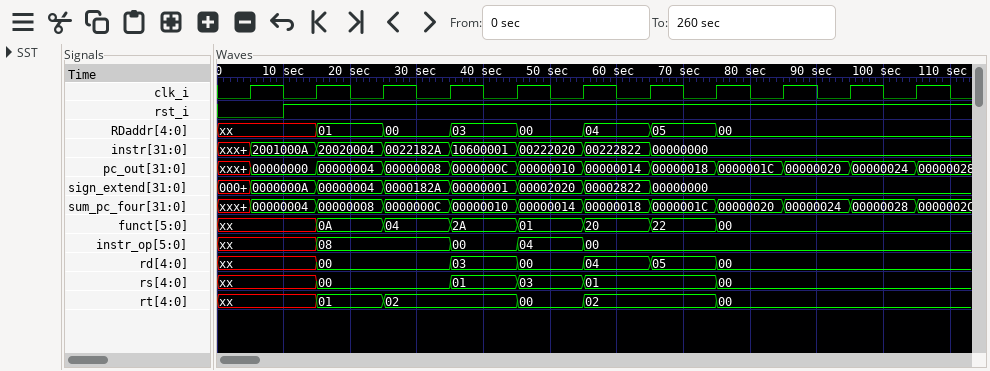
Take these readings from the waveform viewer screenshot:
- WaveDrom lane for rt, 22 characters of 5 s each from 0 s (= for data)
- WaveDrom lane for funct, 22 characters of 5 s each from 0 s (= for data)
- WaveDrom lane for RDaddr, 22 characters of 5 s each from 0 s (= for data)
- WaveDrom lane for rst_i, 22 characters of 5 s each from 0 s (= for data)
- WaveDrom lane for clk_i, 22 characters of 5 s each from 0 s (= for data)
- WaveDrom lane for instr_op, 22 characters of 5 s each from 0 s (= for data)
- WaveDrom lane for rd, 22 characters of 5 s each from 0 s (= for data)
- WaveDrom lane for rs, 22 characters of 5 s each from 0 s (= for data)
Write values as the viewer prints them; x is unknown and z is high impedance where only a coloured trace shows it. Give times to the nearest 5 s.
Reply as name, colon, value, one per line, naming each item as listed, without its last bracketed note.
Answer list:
WaveDrom lane for rt, 22 characters of 5 s each from 0 s: {name: 'rt', wave: 'x..=.=...=.=...=......', data: '01 02 00 02 00'}
WaveDrom lane for funct, 22 characters of 5 s each from 0 s: {name: 'funct', wave: 'x..=.=.=.=.=.=.=......', data: '0A 04 2A 01 20 22 00'}
WaveDrom lane for RDaddr, 22 characters of 5 s each from 0 s: {name: 'RDaddr', wave: 'x..=.=.=.=.=.=.=......', data: '01 00 03 00 04 05 00'}
WaveDrom lane for rst_i, 22 characters of 5 s each from 0 s: {name: 'rst_i', wave: '0.1...................'}
WaveDrom lane for clk_i, 22 characters of 5 s each from 0 s: {name: 'clk_i', wave: '0101010101010101010101'}
WaveDrom lane for instr_op, 22 characters of 5 s each from 0 s: {name: 'instr_op', wave: 'x..=...=.=.=..........', data: '08 00 04 00'}
WaveDrom lane for rd, 22 characters of 5 s each from 0 s: {name: 'rd', wave: 'x..=...=.=.=.=.=......', data: '00 03 00 04 05 00'}
WaveDrom lane for rs, 22 characters of 5 s each from 0 s: {name: 'rs', wave: 'x..=...=.=.=...=......', data: '00 01 03 01 00'}
